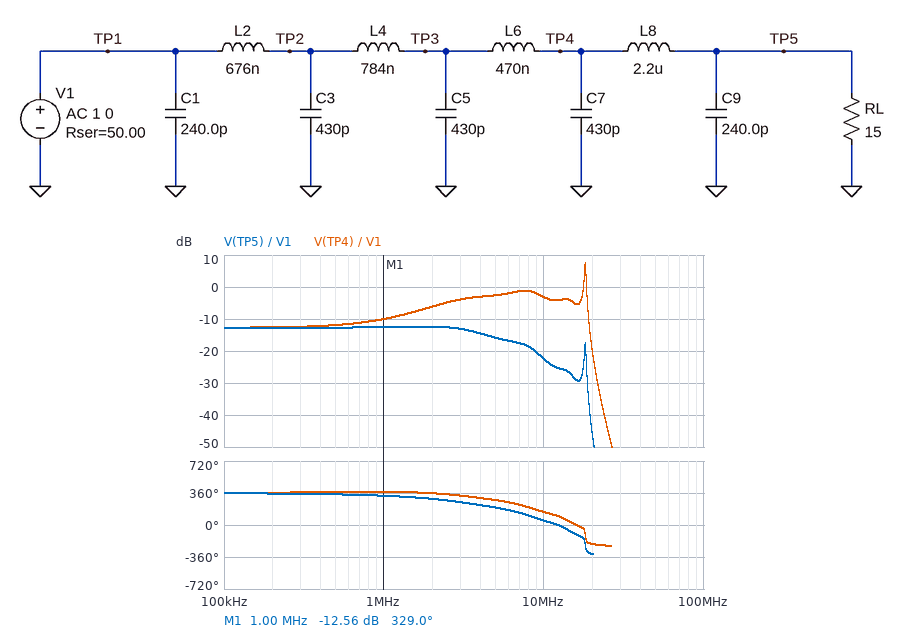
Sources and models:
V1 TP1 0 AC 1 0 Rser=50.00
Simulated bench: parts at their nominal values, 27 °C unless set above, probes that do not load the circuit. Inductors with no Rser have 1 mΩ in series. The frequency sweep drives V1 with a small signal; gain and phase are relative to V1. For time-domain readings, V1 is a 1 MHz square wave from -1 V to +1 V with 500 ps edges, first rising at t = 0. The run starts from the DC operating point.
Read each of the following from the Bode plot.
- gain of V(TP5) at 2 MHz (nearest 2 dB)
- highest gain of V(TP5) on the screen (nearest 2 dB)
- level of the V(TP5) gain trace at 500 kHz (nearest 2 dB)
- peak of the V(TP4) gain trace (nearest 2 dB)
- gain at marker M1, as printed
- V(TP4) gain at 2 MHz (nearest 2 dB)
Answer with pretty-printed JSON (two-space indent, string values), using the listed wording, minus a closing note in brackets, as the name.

{
  "gain of V(TP5) at 2 MHz": "-12 dB",
  "highest gain of V(TP5) on the screen": "-12 dB",
  "level of the V(TP5) gain trace at 500 kHz": "-12 dB",
  "peak of the V(TP4) gain trace": "8 dB",
  "gain at marker M1, as printed": "-12.56 dB",
  "V(TP4) gain at 2 MHz": "-6 dB"
}
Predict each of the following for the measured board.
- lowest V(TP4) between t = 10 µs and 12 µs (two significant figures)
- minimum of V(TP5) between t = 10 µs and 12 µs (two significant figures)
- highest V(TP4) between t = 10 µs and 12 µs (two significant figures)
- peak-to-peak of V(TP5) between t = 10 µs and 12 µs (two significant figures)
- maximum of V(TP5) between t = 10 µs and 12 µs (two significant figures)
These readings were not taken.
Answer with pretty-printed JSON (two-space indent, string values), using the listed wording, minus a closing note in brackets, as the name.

{
  "lowest V(TP4) between t = 10 µs and 12 µs": "-1.2 V",
  "minimum of V(TP5) between t = 10 µs and 12 µs": "-260 mV",
  "highest V(TP4) between t = 10 µs and 12 µs": "1.2 V",
  "peak-to-peak of V(TP5) between t = 10 µs and 12 µs": "520 mV",
  "maximum of V(TP5) between t = 10 µs and 12 µs": "260 mV"
}
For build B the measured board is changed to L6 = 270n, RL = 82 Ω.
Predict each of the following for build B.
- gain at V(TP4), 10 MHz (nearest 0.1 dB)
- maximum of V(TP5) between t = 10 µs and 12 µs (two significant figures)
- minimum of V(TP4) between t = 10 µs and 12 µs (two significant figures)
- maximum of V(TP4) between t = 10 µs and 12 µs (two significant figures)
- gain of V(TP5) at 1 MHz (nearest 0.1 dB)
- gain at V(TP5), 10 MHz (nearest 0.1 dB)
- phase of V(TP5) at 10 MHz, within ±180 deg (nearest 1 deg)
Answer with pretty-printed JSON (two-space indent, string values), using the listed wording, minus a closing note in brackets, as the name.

{
  "gain at V(TP4), 10 MHz": "-4.4 dB",
  "maximum of V(TP5) between t = 10 µs and 12 µs": "700 mV",
  "minimum of V(TP4) between t = 10 µs and 12 µs": "-730 mV",
  "maximum of V(TP4) between t = 10 µs and 12 µs": "730 mV",
  "gain of V(TP5) at 1 MHz": "-4.2 dB",
  "gain at V(TP5), 10 MHz": "-10.5 dB",
  "phase of V(TP5) at 10 MHz, within ±180 deg": "34 deg"
}
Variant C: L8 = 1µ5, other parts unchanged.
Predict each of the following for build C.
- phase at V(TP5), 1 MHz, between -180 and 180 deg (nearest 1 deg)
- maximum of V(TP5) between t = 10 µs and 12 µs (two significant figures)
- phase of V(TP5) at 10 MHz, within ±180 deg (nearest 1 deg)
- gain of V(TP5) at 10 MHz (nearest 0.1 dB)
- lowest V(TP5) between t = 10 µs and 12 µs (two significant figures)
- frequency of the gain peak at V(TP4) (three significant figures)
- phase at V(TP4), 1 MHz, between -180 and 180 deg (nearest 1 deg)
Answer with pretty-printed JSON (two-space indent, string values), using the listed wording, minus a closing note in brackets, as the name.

{
  "phase at V(TP5), 1 MHz, between -180 and 180 deg": "-27 deg",
  "maximum of V(TP5) between t = 10 µs and 12 µs": "270 mV",
  "phase of V(TP5) at 10 MHz, within ±180 deg": "58 deg",
  "gain of V(TP5) at 10 MHz": "-18.8 dB",
  "lowest V(TP5) between t = 10 µs and 12 µs": "-270 mV",
  "frequency of the gain peak at V(TP4)": "18.2 MHz",
  "phase at V(TP4), 1 MHz, between -180 and 180 deg": "6 deg"
}
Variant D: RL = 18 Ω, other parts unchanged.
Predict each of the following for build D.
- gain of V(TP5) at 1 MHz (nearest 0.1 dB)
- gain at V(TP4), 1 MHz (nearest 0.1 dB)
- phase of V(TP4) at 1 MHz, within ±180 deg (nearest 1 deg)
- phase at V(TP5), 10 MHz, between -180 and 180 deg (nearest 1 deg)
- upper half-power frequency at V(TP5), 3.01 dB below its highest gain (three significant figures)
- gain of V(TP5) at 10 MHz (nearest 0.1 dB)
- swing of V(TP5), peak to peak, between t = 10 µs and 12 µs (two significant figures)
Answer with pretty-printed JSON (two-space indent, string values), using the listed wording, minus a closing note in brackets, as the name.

{
  "gain of V(TP5) at 1 MHz": "-11.4 dB",
  "gain at V(TP4), 1 MHz": "-9.5 dB",
  "phase of V(TP4) at 1 MHz, within ±180 deg": "7 deg",
  "phase at V(TP5), 10 MHz, between -180 and 180 deg": "48 deg",
  "upper half-power frequency at V(TP5), 3.01 dB below its highest gain": "4.82 MHz",
  "gain of V(TP5) at 10 MHz": "-21.0 dB",
  "swing of V(TP5), peak to peak, between t = 10 µs and 12 µs": "590 mV"
}
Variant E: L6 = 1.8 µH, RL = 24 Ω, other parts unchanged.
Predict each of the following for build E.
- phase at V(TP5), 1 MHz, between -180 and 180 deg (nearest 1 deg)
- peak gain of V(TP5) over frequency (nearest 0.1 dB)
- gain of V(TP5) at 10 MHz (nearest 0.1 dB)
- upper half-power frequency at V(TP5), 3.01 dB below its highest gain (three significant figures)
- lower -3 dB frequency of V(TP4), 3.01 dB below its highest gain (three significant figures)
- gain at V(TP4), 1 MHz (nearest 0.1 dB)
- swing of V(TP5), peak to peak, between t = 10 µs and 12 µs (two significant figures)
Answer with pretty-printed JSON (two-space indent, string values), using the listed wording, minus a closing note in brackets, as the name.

{
  "phase at V(TP5), 1 MHz, between -180 and 180 deg": "-37 deg",
  "peak gain of V(TP5) over frequency": "-9.8 dB",
  "gain of V(TP5) at 10 MHz": "-16.9 dB",
  "upper half-power frequency at V(TP5), 3.01 dB below its highest gain": "8.71 MHz",
  "lower -3 dB frequency of V(TP4), 3.01 dB below its highest gain": "6.20 MHz",
  "gain at V(TP4), 1 MHz": "-8.7 dB",
  "swing of V(TP5), peak to peak, between t = 10 µs and 12 µs": "740 mV"
}
